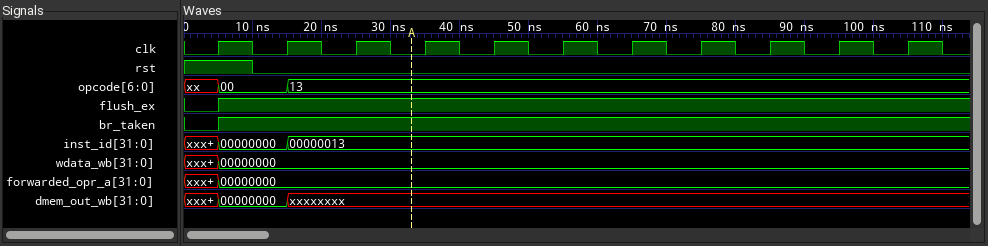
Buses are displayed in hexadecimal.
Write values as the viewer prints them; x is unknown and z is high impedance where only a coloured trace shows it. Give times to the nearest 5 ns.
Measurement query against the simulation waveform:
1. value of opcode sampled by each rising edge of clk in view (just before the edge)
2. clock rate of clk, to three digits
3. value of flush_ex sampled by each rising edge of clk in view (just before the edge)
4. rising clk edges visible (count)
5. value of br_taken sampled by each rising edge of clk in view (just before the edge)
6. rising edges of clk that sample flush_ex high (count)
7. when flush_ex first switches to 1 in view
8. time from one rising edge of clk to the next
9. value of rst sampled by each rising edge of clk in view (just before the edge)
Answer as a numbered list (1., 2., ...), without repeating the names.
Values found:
1. xx, 00, 13, 13, 13, 13, 13, 13, 13, 13, 13
2. 100 MHz
3. 0 1 1 1 1 1 1 1 1 1 1
4. 11
5. 0 1 1 1 1 1 1 1 1 1 1
6. 10
7. 5 ns
8. 10 ns
9. 1 0 0 0 0 0 0 0 0 0 0
